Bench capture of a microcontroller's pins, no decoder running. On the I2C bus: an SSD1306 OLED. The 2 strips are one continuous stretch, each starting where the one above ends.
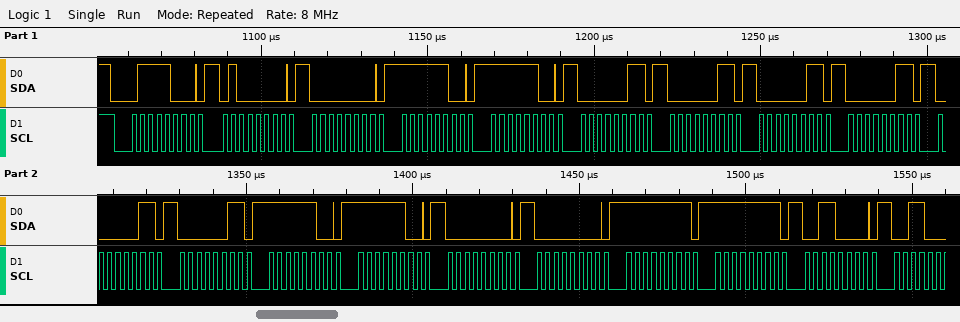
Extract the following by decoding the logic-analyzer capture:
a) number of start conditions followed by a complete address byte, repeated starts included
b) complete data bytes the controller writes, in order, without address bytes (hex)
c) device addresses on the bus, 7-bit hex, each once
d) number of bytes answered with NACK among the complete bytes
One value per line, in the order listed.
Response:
1
40 00 FC FC 03 03 03 03 03 03 FC FC 00 00 FF FF 30
0x3C
0
